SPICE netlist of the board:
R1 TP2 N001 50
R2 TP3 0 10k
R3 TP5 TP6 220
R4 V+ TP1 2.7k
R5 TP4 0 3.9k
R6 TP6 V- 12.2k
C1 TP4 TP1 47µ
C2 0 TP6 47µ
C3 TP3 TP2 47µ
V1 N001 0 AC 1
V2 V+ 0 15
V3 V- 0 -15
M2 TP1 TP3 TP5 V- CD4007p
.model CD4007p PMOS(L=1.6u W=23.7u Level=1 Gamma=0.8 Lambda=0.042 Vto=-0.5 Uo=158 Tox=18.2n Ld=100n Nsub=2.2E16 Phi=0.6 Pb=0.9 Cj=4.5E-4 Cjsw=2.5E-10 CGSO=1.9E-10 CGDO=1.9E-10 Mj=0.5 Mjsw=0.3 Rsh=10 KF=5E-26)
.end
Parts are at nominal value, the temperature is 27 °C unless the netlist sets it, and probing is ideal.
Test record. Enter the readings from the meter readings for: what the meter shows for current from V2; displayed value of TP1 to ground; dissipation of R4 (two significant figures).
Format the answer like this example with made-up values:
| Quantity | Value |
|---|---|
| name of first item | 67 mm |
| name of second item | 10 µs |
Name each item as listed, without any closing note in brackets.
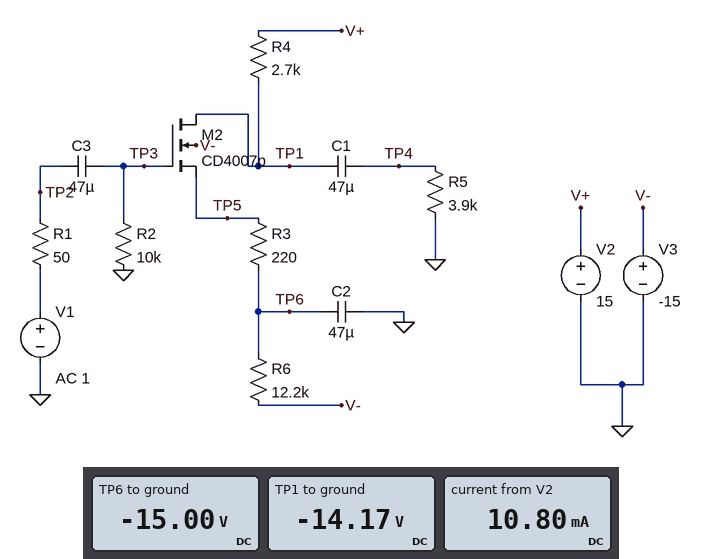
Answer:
| Quantity | Value |
|---|---|
| what the meter shows for current from V2 | 10.80 mA |
| displayed value of TP1 to ground | -14.17 V |
| dissipation of R4 | 320 mW |
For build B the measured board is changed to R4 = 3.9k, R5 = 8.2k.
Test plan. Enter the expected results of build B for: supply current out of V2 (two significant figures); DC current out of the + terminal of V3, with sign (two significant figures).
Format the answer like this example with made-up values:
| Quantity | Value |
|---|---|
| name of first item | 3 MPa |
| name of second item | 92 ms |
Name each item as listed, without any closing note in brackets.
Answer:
| Quantity | Value |
|---|---|
| supply current out of V2 | 7.5 mA |
| DC current out of the + terminal of V3, with sign | -7.5 mA |
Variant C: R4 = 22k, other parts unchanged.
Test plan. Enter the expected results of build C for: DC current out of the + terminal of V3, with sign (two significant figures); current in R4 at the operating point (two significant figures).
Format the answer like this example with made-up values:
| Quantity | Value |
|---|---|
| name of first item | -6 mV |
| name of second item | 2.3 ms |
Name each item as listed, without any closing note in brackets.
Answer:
| Quantity | Value |
|---|---|
| DC current out of the + terminal of V3, with sign | -1.3 mA |
| current in R4 at the operating point | 1.3 mA |
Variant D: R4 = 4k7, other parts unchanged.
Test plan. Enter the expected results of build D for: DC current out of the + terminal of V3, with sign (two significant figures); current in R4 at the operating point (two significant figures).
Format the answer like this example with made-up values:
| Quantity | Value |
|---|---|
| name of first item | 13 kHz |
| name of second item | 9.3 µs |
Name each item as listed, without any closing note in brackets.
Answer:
| Quantity | Value |
|---|---|
| DC current out of the + terminal of V3, with sign | -6.2 mA |
| current in R4 at the operating point | 6.2 mA |
